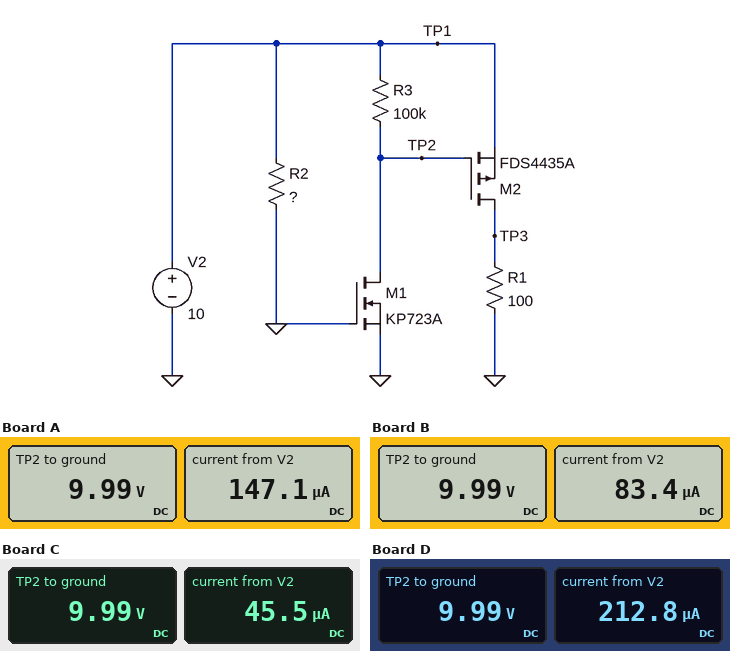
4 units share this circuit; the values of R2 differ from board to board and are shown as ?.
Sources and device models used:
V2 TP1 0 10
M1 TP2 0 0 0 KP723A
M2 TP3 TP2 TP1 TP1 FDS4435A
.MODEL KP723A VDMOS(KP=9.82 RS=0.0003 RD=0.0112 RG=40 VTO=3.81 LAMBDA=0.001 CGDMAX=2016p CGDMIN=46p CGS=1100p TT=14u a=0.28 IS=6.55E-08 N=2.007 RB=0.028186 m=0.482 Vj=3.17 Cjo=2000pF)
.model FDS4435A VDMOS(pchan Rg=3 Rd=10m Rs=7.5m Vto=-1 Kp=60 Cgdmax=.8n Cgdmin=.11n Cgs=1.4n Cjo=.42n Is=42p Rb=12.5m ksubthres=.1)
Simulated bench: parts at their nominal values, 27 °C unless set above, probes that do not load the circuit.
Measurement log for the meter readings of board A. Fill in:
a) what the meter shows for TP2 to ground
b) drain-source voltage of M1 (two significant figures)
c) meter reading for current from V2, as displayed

9.99 V
10 V
147.1 µA
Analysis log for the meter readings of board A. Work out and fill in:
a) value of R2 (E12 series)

68 kΩ
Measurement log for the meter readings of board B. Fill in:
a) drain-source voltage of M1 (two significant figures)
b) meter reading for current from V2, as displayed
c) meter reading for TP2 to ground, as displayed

10 V
83.4 µA
9.99 V
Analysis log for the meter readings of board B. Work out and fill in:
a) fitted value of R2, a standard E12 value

120 kΩ
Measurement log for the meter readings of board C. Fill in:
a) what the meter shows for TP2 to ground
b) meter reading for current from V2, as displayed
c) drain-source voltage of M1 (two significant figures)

9.99 V
45.5 µA
10 V
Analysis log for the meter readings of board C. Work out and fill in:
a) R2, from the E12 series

220 kΩ
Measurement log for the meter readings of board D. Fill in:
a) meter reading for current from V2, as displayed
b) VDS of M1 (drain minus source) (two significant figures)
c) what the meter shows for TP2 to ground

212.8 µA
10 V
9.99 V
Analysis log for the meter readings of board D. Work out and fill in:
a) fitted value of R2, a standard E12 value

47 kΩ
